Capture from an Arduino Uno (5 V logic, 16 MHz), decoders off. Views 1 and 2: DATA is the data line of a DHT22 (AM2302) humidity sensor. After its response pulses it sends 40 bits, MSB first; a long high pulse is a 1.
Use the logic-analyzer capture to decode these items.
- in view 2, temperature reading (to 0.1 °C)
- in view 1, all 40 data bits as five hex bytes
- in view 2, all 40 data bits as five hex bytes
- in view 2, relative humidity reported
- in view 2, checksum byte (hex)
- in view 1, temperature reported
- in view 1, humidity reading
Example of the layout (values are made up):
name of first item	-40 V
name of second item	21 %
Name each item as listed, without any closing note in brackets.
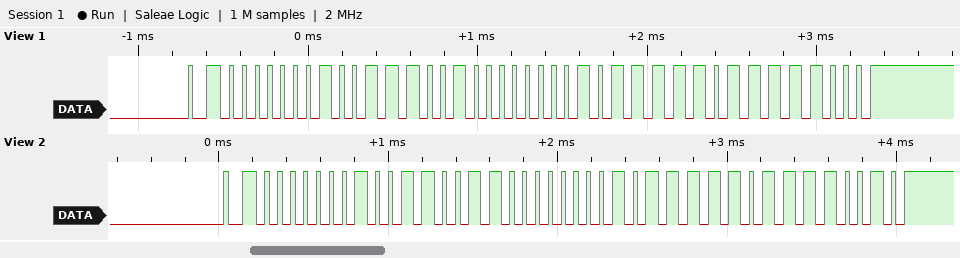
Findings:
in view 2, temperature reading	19.0 °C
in view 1, all 40 data bits as five hex bytes	01 39 00 BE F8
in view 2, all 40 data bits as five hex bytes	01 33 00 BE F2
in view 2, relative humidity reported	30.7 %
in view 2, checksum byte	0xF2
in view 1, temperature reported	19.0 °C
in view 1, humidity reading	31.3 %
